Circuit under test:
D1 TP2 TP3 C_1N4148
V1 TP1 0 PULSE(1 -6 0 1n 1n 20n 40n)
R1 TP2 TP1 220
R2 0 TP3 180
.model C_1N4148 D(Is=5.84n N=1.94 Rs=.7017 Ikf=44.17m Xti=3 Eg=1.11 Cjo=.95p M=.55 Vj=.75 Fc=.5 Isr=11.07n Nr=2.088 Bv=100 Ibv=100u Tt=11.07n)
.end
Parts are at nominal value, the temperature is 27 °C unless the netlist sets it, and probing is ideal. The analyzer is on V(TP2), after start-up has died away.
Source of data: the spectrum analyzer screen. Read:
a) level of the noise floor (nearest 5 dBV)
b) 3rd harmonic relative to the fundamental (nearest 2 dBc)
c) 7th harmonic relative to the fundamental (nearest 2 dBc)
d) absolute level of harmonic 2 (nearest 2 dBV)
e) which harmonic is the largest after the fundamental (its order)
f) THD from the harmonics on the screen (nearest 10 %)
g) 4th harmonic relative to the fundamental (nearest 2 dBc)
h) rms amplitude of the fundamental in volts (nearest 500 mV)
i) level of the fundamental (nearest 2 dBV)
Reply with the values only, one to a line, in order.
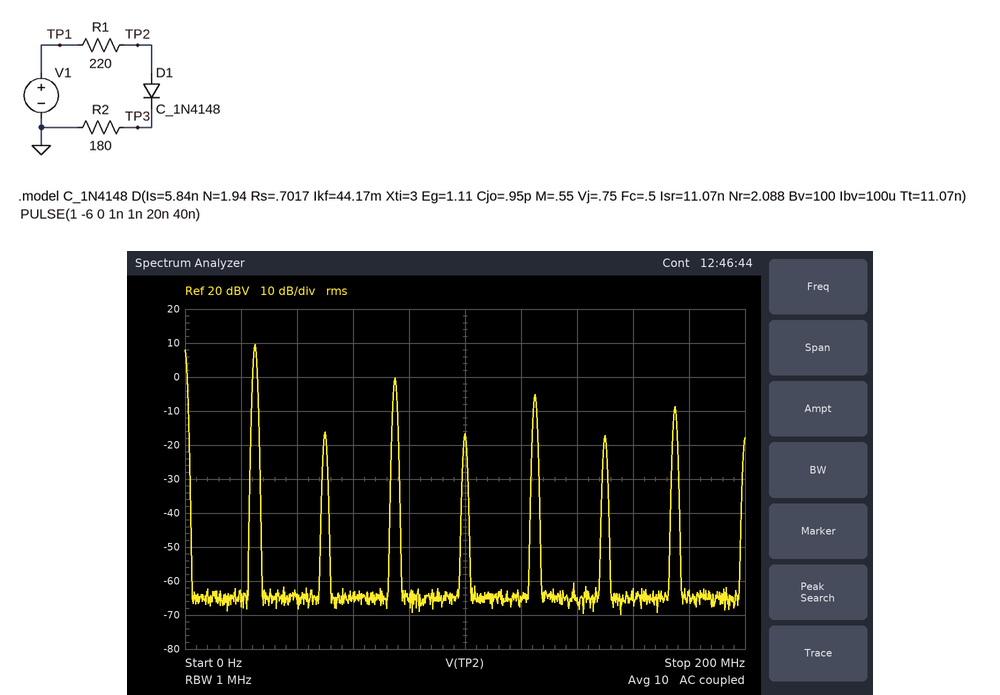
-65 dBV
-10 dBc
-18 dBc
-16 dBV
3
40 %
-26 dBc
3.0 V
10 dBV
